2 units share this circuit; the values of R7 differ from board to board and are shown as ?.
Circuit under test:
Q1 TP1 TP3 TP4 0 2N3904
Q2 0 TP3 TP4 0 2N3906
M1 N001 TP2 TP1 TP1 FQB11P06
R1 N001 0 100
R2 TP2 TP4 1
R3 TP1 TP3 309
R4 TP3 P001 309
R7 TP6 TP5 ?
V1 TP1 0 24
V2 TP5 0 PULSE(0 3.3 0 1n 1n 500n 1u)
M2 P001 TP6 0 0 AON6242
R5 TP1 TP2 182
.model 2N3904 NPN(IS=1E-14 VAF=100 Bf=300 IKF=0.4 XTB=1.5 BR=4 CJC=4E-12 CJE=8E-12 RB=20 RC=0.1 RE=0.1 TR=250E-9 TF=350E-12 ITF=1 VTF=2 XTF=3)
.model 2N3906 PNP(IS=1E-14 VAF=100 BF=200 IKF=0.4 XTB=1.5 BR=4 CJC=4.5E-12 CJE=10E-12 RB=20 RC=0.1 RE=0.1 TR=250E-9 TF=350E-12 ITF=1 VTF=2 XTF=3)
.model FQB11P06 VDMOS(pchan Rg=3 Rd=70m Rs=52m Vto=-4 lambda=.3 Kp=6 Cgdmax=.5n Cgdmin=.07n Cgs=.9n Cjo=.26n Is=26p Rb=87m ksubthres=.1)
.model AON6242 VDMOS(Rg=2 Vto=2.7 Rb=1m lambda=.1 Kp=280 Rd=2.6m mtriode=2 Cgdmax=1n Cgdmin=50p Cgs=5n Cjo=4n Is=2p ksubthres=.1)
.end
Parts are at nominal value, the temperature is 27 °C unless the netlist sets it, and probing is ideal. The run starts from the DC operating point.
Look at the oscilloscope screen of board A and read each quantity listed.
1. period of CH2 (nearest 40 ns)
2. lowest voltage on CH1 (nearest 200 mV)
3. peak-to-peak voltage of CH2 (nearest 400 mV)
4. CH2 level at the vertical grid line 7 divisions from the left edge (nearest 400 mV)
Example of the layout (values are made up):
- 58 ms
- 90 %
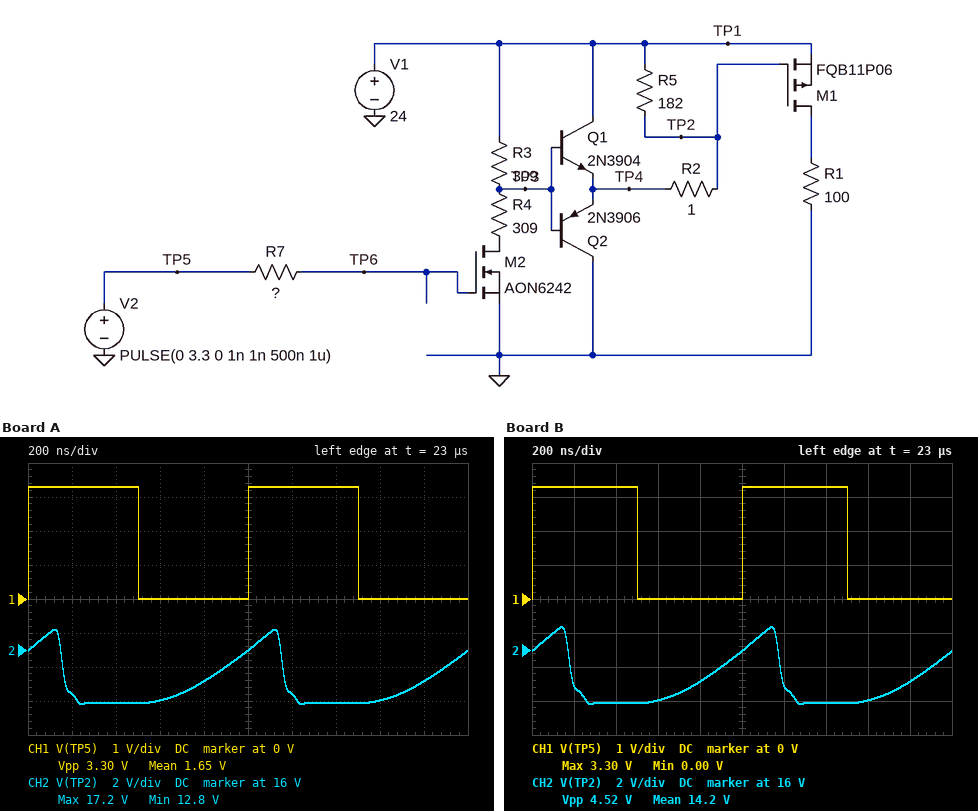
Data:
- 1.00 µs
- 0 V
- 4.4 V
- 12.8 V
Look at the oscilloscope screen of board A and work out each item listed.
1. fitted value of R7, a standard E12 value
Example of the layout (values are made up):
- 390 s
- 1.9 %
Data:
- 15 Ω
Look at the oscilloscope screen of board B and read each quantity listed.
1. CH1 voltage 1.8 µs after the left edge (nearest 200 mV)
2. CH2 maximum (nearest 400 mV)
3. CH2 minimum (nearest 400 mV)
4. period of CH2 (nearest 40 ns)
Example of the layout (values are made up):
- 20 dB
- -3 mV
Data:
- 0 V
- 17.2 V
- 12.8 V
- 1.00 µs
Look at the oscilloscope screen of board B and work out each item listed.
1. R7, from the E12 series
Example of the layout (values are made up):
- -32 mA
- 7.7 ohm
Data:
- 18 Ω
